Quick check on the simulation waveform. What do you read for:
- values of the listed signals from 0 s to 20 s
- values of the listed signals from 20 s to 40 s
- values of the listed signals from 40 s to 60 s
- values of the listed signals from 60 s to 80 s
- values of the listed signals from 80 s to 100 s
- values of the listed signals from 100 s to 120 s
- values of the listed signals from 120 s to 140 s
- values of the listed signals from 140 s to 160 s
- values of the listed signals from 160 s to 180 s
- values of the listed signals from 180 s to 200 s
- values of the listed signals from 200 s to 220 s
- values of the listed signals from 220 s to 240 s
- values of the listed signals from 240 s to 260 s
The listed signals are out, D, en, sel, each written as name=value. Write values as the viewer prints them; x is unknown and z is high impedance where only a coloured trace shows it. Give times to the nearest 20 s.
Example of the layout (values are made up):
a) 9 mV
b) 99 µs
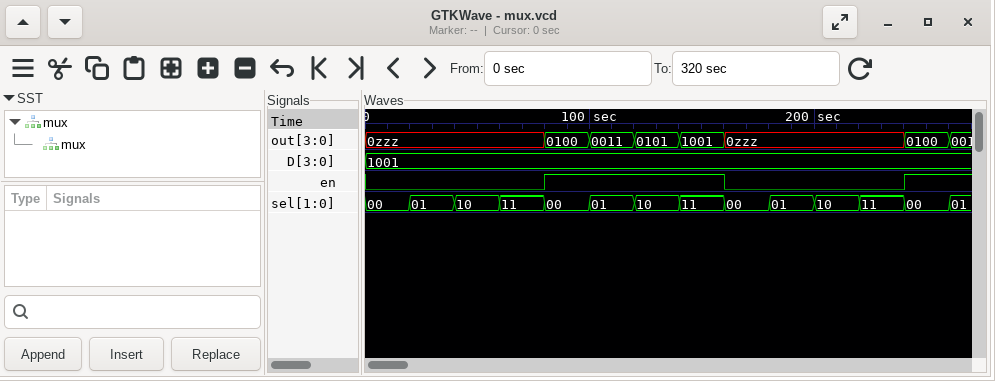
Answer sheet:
a) out=0zzz, D=1001, en=0, sel=00
b) out=0zzz, D=1001, en=0, sel=01
c) out=0zzz, D=1001, en=0, sel=10
d) out=0zzz, D=1001, en=0, sel=11
e) out=0100, D=1001, en=1, sel=00
f) out=0011, D=1001, en=1, sel=01
g) out=0101, D=1001, en=1, sel=10
h) out=1001, D=1001, en=1, sel=11
i) out=0zzz, D=1001, en=0, sel=00
j) out=0zzz, D=1001, en=0, sel=01
k) out=0zzz, D=1001, en=0, sel=10
l) out=0zzz, D=1001, en=0, sel=11
m) out=0100, D=1001, en=1, sel=00
